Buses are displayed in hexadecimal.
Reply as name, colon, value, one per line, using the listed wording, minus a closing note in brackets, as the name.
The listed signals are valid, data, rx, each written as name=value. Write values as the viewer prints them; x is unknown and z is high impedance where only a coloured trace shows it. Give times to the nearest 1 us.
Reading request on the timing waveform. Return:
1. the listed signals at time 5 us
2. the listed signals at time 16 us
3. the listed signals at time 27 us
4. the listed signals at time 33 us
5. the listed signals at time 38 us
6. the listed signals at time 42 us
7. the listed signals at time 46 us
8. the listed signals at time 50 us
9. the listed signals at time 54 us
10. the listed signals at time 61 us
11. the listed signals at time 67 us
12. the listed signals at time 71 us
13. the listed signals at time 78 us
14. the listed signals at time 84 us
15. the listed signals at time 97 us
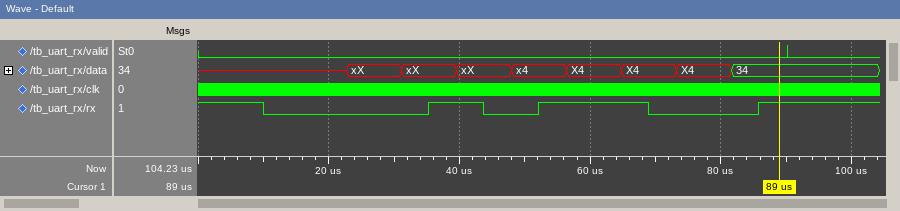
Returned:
the listed signals at time 5 us: valid=0, data=x, rx=1
the listed signals at time 16 us: valid=0, data=x, rx=0
the listed signals at time 27 us: valid=0, data=xX, rx=0
the listed signals at time 33 us: valid=0, data=xX, rx=0
the listed signals at time 38 us: valid=0, data=xX, rx=1
the listed signals at time 42 us: valid=0, data=xX, rx=1
the listed signals at time 46 us: valid=0, data=xX, rx=0
the listed signals at time 50 us: valid=0, data=x4, rx=0
the listed signals at time 54 us: valid=0, data=x4, rx=1
the listed signals at time 61 us: valid=0, data=X4, rx=1
the listed signals at time 67 us: valid=0, data=X4, rx=1
the listed signals at time 71 us: valid=0, data=X4, rx=0
the listed signals at time 78 us: valid=0, data=X4, rx=0
the listed signals at time 84 us: valid=0, data=34, rx=0
the listed signals at time 97 us: valid=0, data=34, rx=1
